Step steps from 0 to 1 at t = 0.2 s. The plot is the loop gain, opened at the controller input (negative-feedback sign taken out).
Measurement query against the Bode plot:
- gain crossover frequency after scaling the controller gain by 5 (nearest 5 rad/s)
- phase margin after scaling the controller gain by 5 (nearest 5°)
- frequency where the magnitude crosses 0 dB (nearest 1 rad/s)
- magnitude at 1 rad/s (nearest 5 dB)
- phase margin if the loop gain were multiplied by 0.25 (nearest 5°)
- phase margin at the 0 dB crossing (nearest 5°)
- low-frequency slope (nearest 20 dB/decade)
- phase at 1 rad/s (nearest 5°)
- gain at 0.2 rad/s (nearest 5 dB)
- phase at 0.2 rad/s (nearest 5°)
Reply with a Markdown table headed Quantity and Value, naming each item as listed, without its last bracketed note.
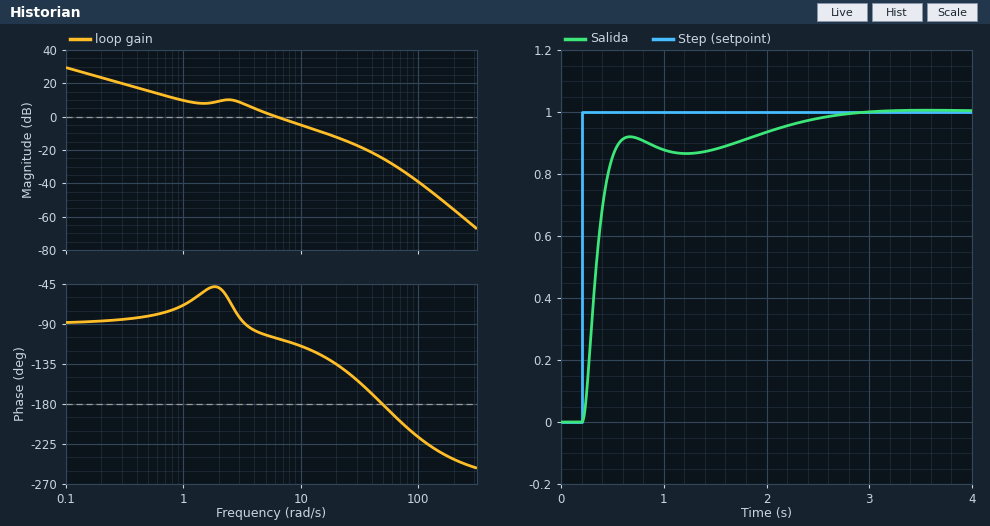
| Quantity | Value |
|---|---|
| gain crossover frequency after scaling the controller gain by 5 | 25 rad/s |
| phase margin after scaling the controller gain by 5 | 40° |
| frequency where the magnitude crosses 0 dB | 6 rad/s |
| magnitude at 1 rad/s | 10 dB |
| phase margin if the loop gain were multiplied by 0.25 | 105° |
| phase margin at the 0 dB crossing | 75° |
| low-frequency slope | -20 dB/decade |
| phase at 1 rad/s | -70° |
| gain at 0.2 rad/s | 25 dB |
| phase at 0.2 rad/s | -85° |
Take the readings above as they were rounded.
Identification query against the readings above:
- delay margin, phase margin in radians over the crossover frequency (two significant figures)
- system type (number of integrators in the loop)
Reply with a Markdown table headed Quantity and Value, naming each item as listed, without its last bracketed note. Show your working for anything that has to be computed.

| Quantity | Value |
|---|---|
| delay margin, phase margin in radians over the crossover frequency | 75 × π / 180 / 6 = 0.22 s |
| system type | 1 |
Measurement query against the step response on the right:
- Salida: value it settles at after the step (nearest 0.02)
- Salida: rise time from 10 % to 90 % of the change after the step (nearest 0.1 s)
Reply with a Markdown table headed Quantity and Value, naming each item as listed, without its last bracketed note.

| Quantity | Value |
|---|---|
| Salida: value it settles at after the step | 1.00 |
| Salida: rise time from 10 % to 90 % of the change after the step | 0.3 s |
